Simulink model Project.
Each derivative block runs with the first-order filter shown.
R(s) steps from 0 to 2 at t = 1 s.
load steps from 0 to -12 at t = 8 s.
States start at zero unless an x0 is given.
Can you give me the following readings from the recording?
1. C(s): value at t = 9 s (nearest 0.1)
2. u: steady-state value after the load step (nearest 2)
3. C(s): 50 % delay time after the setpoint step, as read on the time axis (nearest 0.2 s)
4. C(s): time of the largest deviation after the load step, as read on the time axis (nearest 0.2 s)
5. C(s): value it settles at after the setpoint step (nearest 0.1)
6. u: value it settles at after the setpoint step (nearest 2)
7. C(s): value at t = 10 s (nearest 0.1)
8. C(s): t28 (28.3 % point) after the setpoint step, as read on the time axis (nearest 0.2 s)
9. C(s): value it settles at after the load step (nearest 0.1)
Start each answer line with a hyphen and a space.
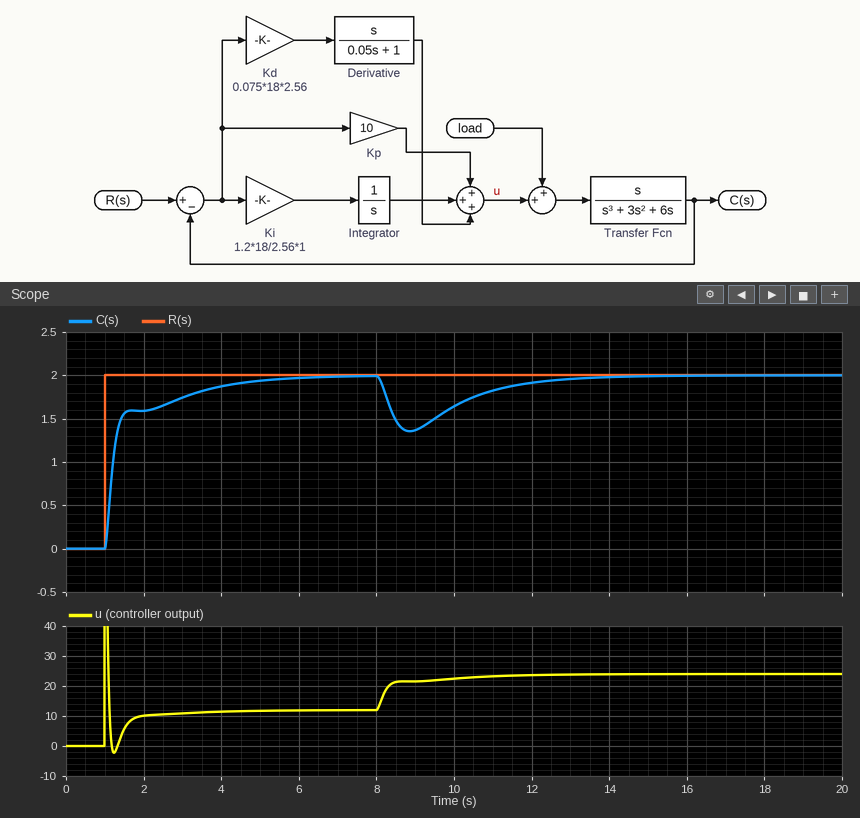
- 1.4
- 24
- 1.2 s
- 8.8 s
- 2.0
- 12
- 1.6
- 1.2 s
- 2.0
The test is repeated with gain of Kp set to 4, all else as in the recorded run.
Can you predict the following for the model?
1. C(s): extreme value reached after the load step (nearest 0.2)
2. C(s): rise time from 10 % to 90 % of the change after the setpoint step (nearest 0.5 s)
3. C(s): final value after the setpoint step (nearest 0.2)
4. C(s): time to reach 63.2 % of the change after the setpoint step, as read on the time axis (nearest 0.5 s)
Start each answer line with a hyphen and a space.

- 1.2
- 2.0 s
- 2.0
- 1.5 s
